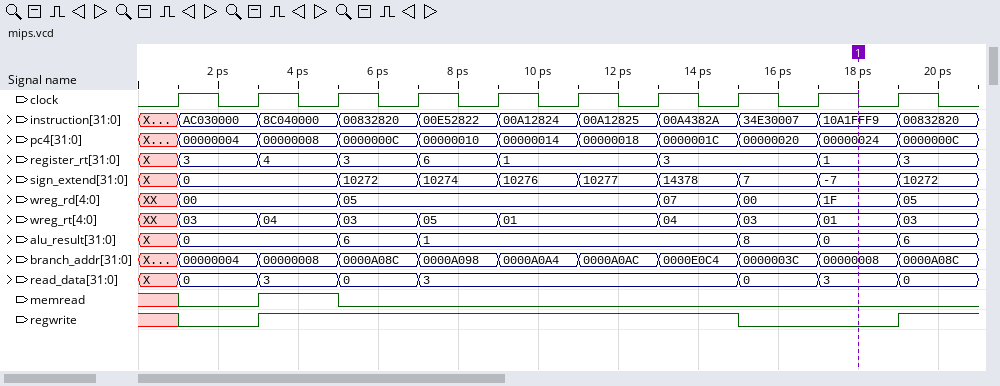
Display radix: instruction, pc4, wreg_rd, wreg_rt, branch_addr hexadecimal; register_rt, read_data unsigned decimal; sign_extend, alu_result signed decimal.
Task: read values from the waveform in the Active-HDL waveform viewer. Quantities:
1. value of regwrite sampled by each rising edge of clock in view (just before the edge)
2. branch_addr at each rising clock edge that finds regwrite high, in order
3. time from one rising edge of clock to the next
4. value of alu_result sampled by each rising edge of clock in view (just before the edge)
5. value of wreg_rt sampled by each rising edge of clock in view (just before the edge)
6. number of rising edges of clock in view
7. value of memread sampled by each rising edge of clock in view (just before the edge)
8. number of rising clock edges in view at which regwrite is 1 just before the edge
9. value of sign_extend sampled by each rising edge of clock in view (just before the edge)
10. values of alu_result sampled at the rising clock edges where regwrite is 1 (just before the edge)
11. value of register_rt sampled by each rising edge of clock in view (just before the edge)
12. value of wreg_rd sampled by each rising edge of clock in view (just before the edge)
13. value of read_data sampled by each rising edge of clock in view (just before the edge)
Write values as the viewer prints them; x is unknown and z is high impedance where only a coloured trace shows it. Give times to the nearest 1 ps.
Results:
x 0 1 1 1 1 1 1 0 0
00000008, 0000A08C, 0000A098, 0000A0A4, 0000A0AC, 0000E0C4
2 ps
X, 0, 0, 6, 1, 1, 1, 1, 8, 0
XX, 03, 04, 03, 05, 01, 01, 04, 03, 01
10
x 0 1 0 0 0 0 0 0 0
6
X, 0, 0, 10272, 10274, 10276, 10277, 14378, 7, -7
0, 6, 1, 1, 1, 1
X, 3, 4, 3, 6, 1, 1, 3, 3, 1
XX, 00, 00, 05, 05, 05, 05, 07, 00, 1F
X, 0, 3, 0, 3, 3, 3, 3, 0, 3
